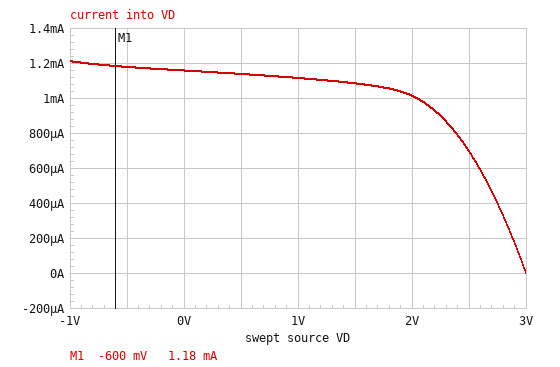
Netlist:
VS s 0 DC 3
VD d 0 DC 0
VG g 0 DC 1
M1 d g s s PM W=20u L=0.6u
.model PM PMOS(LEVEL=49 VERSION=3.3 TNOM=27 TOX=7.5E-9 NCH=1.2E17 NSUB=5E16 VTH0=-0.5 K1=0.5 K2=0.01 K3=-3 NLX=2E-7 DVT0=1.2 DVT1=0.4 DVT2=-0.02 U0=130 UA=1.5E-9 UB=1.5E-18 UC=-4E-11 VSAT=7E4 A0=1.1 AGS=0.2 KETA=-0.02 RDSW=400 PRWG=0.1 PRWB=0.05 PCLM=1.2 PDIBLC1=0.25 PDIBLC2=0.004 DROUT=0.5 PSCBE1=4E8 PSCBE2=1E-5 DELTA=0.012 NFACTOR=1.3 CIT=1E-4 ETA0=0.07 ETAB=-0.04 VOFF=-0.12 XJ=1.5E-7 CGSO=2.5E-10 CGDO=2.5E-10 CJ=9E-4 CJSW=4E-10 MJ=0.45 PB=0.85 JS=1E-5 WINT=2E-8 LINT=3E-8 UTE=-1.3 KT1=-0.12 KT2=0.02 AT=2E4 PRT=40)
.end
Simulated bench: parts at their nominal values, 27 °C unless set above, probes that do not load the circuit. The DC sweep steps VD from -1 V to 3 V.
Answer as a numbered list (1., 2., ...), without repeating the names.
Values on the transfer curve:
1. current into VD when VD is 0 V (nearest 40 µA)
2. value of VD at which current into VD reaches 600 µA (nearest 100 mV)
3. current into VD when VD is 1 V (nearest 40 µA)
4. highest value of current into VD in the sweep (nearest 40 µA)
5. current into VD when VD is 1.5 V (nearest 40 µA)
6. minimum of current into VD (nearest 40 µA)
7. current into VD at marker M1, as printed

1. 1.16 mA
2. 2.6 V
3. 1.12 mA
4. 1.20 mA
5. 1.08 mA
6. 0 A
7. 1.18 mA
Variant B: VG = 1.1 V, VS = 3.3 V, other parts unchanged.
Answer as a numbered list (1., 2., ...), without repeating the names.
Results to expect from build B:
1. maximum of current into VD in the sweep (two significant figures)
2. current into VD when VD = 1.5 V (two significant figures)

1. 1.5 mA
2. 1.3 mA
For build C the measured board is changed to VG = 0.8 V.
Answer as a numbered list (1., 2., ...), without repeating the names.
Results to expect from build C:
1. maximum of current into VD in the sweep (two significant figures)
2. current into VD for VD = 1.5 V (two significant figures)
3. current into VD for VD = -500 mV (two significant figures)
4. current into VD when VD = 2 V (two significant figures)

1. 1.5 mA
2. 1.3 mA
3. 1.4 mA
4. 1.2 mA
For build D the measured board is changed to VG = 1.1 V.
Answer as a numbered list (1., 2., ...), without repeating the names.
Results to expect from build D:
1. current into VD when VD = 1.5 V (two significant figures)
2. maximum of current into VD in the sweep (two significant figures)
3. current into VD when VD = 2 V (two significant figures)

1. 970 µA
2. 1.1 mA
3. 920 µA
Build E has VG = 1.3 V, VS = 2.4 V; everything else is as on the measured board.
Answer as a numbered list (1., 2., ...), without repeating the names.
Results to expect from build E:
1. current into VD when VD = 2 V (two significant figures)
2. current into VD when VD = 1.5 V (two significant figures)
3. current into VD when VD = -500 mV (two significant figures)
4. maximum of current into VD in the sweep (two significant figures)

1. 190 µA
2. 210 µA
3. 240 µA
4. 250 µA
